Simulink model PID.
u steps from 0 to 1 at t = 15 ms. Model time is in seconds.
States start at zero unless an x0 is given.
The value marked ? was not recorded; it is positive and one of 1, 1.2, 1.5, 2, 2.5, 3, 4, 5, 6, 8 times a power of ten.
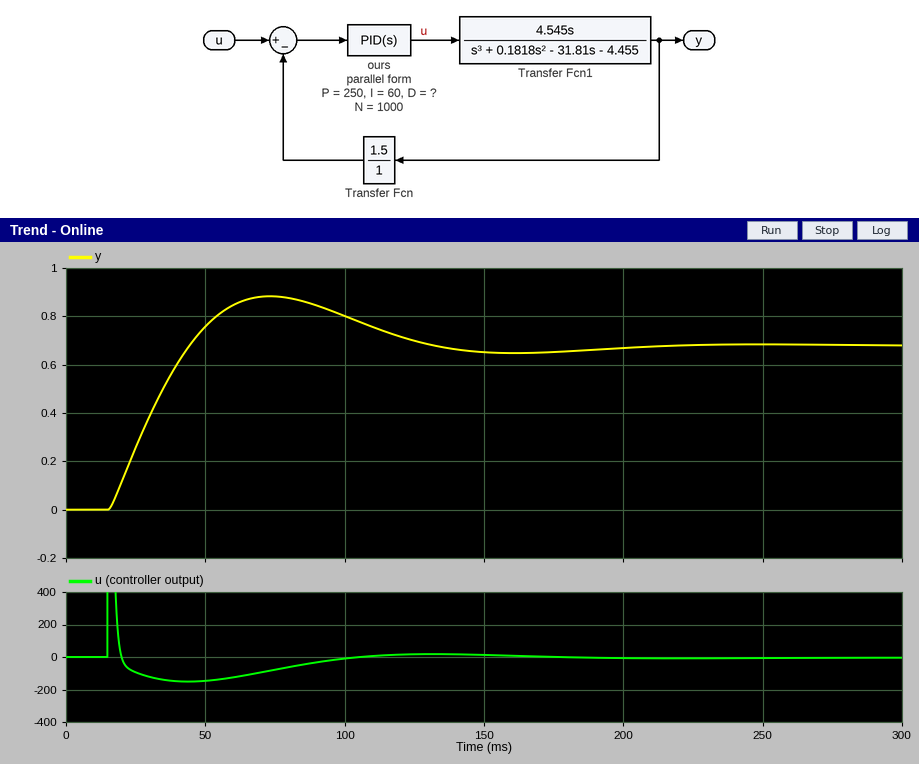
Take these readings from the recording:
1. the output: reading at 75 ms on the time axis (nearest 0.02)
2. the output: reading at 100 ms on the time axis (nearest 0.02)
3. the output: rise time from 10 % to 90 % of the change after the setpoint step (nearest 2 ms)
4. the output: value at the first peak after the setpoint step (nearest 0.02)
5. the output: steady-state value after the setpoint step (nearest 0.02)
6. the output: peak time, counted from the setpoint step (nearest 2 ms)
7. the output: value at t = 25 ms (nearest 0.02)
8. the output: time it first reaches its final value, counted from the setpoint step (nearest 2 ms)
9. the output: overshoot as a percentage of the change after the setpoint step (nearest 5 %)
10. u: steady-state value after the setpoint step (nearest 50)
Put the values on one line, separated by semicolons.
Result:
0.88; 0.80; 22 ms; 0.88; 0.68; 58 ms; 0.26; 30 ms; 30 %; 0
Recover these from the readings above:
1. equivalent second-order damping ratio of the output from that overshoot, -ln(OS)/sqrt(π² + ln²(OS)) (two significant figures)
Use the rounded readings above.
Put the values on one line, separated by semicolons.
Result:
0.36
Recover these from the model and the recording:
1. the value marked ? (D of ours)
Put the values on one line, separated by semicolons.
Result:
6
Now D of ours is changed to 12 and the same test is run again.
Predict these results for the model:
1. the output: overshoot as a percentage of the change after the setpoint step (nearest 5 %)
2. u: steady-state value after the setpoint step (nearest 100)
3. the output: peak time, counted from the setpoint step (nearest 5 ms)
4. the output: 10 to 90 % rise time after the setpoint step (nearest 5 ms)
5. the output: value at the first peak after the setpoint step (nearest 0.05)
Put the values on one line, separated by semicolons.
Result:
15 %; 0; 45 ms; 15 ms; 0.75
